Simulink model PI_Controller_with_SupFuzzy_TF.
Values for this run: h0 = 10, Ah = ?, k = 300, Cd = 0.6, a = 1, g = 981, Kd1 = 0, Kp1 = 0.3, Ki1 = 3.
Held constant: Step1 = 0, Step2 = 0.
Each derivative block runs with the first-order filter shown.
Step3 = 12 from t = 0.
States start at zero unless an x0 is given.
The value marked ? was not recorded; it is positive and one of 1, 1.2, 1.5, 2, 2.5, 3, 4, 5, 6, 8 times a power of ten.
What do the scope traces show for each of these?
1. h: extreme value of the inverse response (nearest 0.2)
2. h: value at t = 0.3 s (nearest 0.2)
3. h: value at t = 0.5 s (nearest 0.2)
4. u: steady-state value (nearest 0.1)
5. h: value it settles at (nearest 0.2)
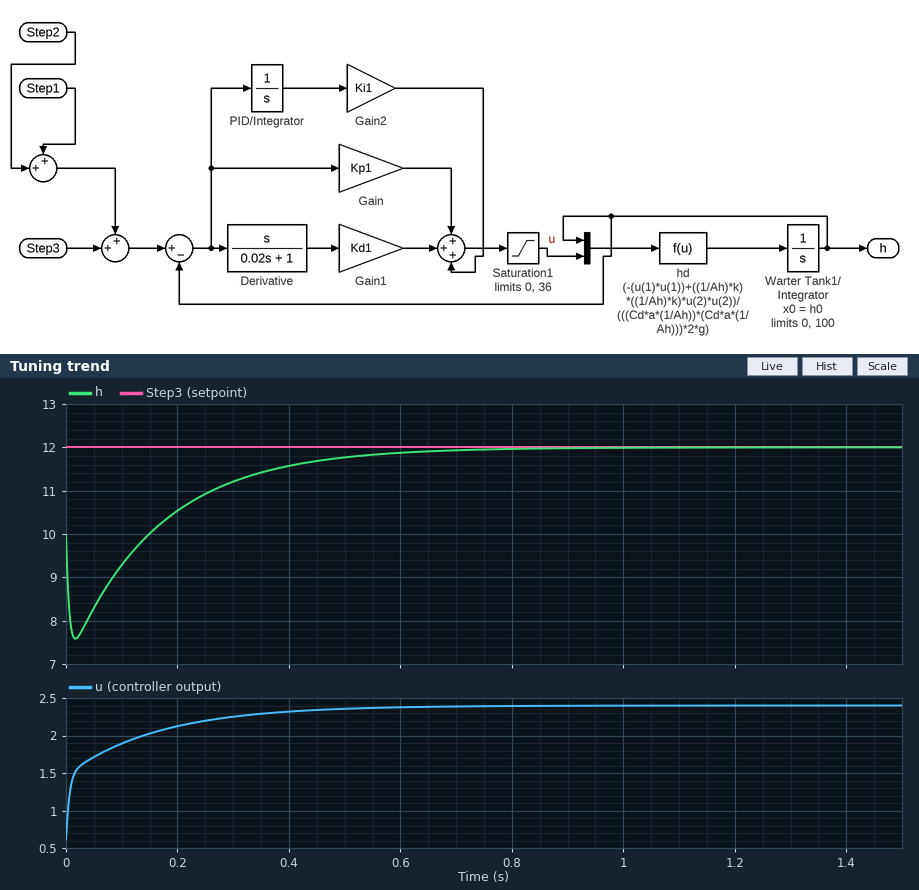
7.6
11.2
11.8
2.4
12.0
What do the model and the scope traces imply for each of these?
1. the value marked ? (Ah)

60
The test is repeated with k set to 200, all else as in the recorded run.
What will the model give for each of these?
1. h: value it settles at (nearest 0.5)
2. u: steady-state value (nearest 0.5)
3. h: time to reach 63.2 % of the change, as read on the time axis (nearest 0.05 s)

12.0
3.5
0.40 s
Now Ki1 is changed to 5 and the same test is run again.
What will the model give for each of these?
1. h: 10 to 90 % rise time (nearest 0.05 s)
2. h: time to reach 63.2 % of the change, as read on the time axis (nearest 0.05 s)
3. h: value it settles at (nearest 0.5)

0.20 s
0.20 s
12.0
